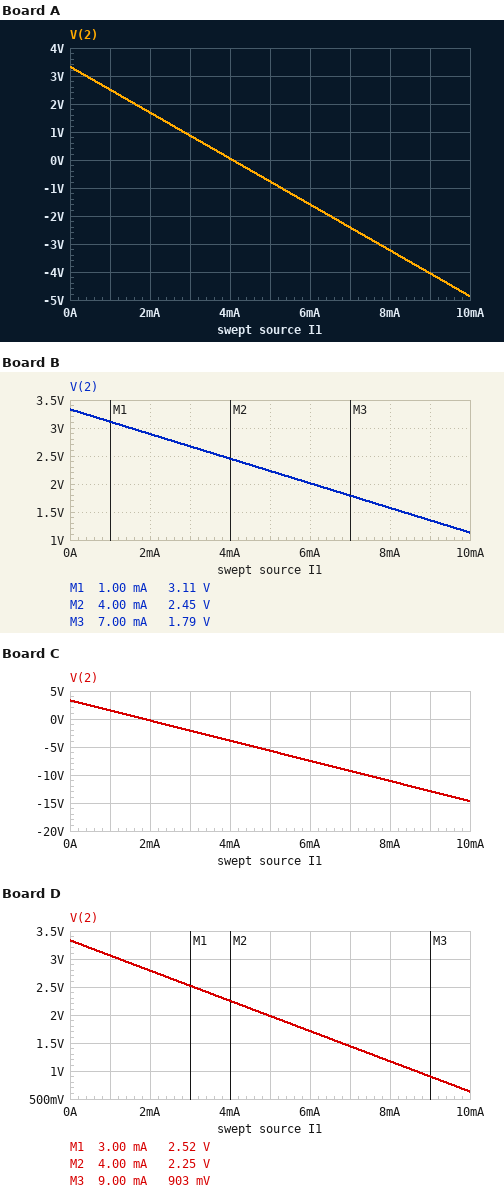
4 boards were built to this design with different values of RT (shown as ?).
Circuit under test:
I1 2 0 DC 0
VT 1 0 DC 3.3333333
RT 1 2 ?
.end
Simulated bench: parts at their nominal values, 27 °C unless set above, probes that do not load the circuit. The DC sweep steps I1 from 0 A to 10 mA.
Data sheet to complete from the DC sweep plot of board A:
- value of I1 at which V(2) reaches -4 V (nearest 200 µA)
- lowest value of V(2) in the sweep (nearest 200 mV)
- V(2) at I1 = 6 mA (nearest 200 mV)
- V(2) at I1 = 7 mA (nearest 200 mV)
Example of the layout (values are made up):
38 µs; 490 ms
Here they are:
9.0 mA; -4.8 V; -1.6 V; -2.4 V
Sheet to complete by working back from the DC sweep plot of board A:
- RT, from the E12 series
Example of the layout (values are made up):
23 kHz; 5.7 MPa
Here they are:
820 Ω
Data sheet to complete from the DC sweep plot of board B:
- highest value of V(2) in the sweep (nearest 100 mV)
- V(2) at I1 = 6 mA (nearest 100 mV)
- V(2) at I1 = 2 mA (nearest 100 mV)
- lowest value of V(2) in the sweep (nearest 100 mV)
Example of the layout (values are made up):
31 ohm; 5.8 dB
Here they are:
3.3 V; 2.0 V; 2.9 V; 1.1 V
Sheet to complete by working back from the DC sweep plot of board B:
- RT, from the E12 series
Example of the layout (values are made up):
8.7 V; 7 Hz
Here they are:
220 Ω
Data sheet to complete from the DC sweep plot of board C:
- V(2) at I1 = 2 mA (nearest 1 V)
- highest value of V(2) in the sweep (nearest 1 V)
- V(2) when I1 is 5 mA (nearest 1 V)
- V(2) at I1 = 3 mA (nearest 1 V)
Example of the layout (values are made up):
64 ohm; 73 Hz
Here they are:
0 V; 3 V; -6 V; -2 V
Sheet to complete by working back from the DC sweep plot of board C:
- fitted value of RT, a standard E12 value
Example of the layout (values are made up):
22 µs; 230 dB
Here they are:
1.8 kΩ
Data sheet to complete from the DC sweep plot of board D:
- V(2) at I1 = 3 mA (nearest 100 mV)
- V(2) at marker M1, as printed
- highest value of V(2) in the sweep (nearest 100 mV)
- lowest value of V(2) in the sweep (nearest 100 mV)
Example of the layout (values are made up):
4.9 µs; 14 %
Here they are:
2.5 V; 2.52 V; 3.3 V; 600 mV
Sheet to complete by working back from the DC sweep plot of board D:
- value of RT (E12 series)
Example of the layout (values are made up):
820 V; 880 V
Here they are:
270 Ω
